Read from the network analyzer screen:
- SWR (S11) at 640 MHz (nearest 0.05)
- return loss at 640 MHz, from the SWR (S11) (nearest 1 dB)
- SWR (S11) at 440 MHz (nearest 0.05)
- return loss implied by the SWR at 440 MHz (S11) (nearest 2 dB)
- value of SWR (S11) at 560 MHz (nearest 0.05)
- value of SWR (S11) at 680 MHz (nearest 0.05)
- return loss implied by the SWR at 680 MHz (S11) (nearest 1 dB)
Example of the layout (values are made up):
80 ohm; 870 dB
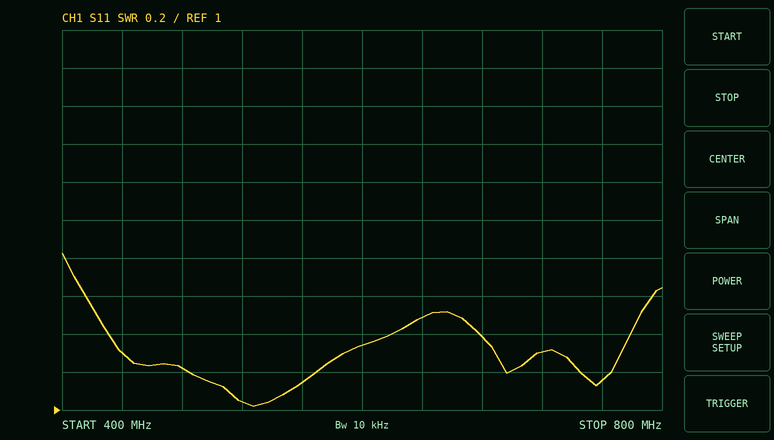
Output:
1.50; 14 dB; 1.30; 18 dB; 1.15; 1.40; 16 dB
